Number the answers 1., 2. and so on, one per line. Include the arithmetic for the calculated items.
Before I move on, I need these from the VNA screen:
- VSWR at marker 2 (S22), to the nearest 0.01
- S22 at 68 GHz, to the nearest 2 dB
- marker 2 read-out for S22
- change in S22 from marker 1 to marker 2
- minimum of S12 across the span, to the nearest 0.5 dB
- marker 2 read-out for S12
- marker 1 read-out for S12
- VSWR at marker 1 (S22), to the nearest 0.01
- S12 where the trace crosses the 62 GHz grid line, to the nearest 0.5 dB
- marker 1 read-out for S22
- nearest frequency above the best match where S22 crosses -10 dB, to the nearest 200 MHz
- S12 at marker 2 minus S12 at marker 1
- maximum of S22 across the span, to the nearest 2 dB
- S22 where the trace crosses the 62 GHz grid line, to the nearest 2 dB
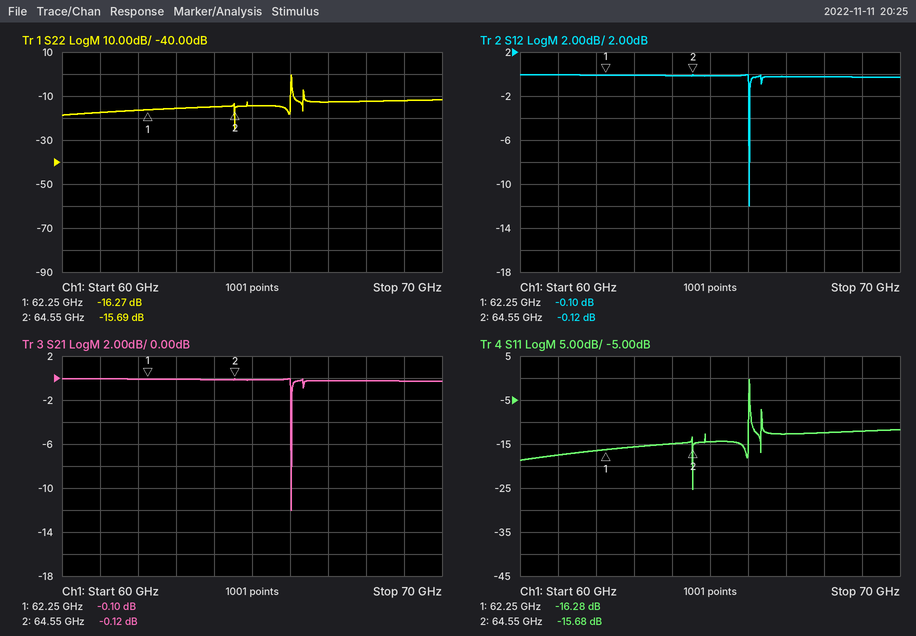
1. (1 + 0.1642)/(1 − 0.1642) ≈ 1.39
2. -12 dB
3. -15.69 dB
4. -15.69 − (-16.27) = 0.58 dB
5. -12.0 dB
6. -0.12 dB
7. -0.10 dB
8. (1 + 0.1536)/(1 − 0.1536) ≈ 1.36
9. 0.0 dB
10. -16.27 dB
11. 66.0 GHz
12. -0.12 − (-0.1) = -0.02 dB
13. 0 dB
14. -16 dB
